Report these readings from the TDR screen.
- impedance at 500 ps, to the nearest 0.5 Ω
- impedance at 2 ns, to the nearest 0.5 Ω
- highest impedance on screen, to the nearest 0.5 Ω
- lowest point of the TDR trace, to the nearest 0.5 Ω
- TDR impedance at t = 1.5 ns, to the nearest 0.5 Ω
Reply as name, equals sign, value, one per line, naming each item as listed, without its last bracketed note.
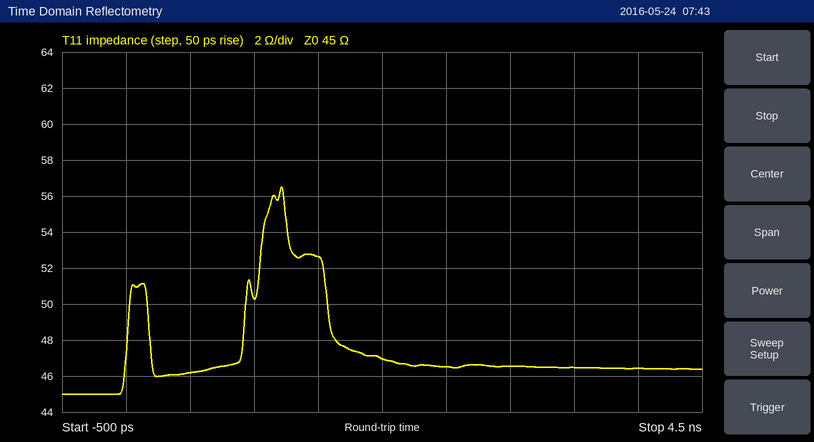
impedance at 500 ps, to the nearest 0.5 Ω = 46.0 Ω
impedance at 2 ns, to the nearest 0.5 Ω = 47.0 Ω
highest impedance on screen, to the nearest 0.5 Ω = 56.5 Ω
lowest point of the TDR trace, to the nearest 0.5 Ω = 45.0 Ω
TDR impedance at t = 1.5 ns, to the nearest 0.5 Ω = 52.5 Ω
